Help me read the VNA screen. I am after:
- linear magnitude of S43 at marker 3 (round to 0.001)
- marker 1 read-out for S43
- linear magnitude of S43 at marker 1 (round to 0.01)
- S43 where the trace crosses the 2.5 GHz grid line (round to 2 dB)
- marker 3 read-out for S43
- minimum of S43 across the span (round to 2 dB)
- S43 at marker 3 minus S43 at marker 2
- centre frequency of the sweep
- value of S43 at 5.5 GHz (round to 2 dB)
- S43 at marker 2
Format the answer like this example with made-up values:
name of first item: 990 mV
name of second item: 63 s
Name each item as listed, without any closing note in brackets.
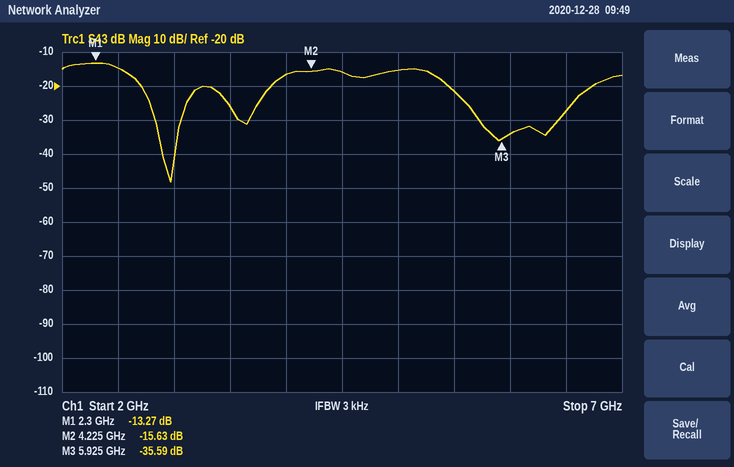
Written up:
linear magnitude of S43 at marker 3: 0.017
marker 1 read-out for S43: -13.27 dB
linear magnitude of S43 at marker 1: 0.22
S43 where the trace crosses the 2.5 GHz grid line: -14 dB
marker 3 read-out for S43: -35.59 dB
minimum of S43 across the span: -48 dB
S43 at marker 3 minus S43 at marker 2: -19.96 dB
centre frequency of the sweep: 4.5 GHz
value of S43 at 5.5 GHz: -22 dB
S43 at marker 2: -15.63 dB
